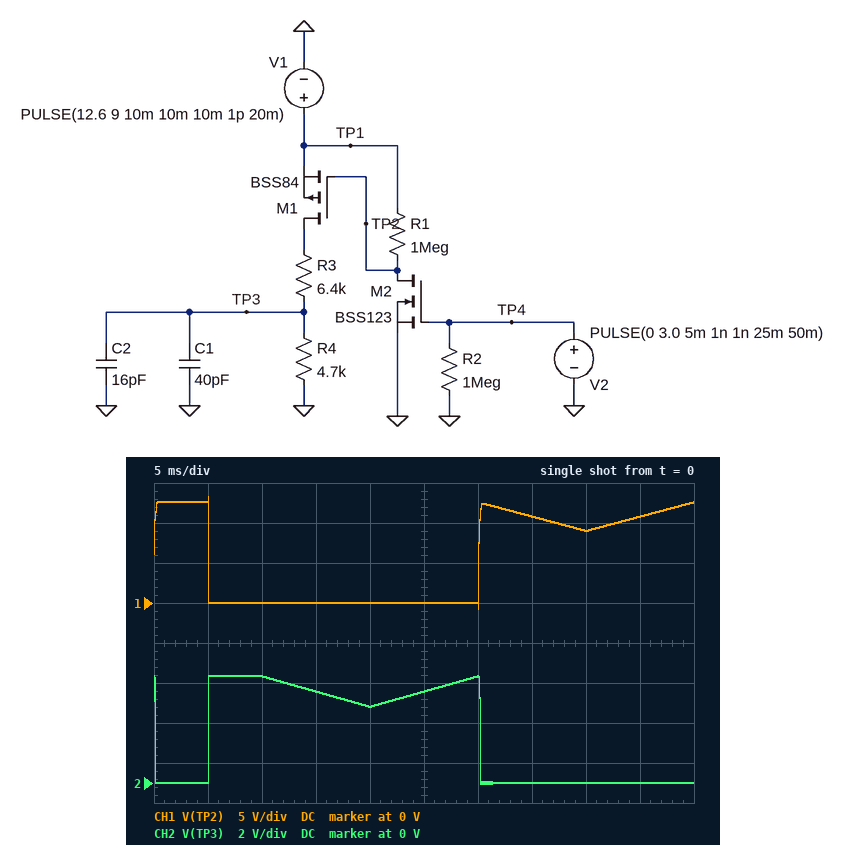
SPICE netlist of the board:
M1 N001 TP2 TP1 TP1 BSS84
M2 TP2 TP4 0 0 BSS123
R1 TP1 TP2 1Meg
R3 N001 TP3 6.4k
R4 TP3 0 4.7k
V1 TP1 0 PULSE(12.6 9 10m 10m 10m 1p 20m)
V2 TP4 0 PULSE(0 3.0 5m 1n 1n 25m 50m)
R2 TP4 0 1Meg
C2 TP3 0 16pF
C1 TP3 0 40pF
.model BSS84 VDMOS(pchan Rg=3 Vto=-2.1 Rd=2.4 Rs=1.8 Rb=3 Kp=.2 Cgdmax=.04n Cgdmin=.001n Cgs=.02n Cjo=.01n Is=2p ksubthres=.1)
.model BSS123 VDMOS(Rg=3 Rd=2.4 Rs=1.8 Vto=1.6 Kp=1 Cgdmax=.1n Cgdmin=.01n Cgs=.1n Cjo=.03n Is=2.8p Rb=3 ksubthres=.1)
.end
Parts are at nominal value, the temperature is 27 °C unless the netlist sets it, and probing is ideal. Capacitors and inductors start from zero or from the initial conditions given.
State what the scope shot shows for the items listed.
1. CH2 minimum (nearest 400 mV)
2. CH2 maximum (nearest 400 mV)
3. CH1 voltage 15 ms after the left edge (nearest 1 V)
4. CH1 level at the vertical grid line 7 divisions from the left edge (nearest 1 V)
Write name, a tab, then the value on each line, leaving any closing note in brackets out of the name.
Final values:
CH2 minimum	0 V
CH2 maximum	5.2 V
CH1 voltage 15 ms after the left edge	0 V
CH1 level at the vertical grid line 7 divisions from the left edge	11 V
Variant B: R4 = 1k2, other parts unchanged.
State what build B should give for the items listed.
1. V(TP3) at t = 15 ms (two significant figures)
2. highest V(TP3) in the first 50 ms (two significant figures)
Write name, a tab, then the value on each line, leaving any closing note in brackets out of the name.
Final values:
V(TP3) at t = 15 ms	1.7 V
highest V(TP3) in the first 50 ms	2.0 V
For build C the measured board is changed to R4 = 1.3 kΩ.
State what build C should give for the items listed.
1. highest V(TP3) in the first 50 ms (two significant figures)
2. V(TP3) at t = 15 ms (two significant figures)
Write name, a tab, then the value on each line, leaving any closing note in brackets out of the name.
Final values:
highest V(TP3) in the first 50 ms	2.1 V
V(TP3) at t = 15 ms	1.8 V
